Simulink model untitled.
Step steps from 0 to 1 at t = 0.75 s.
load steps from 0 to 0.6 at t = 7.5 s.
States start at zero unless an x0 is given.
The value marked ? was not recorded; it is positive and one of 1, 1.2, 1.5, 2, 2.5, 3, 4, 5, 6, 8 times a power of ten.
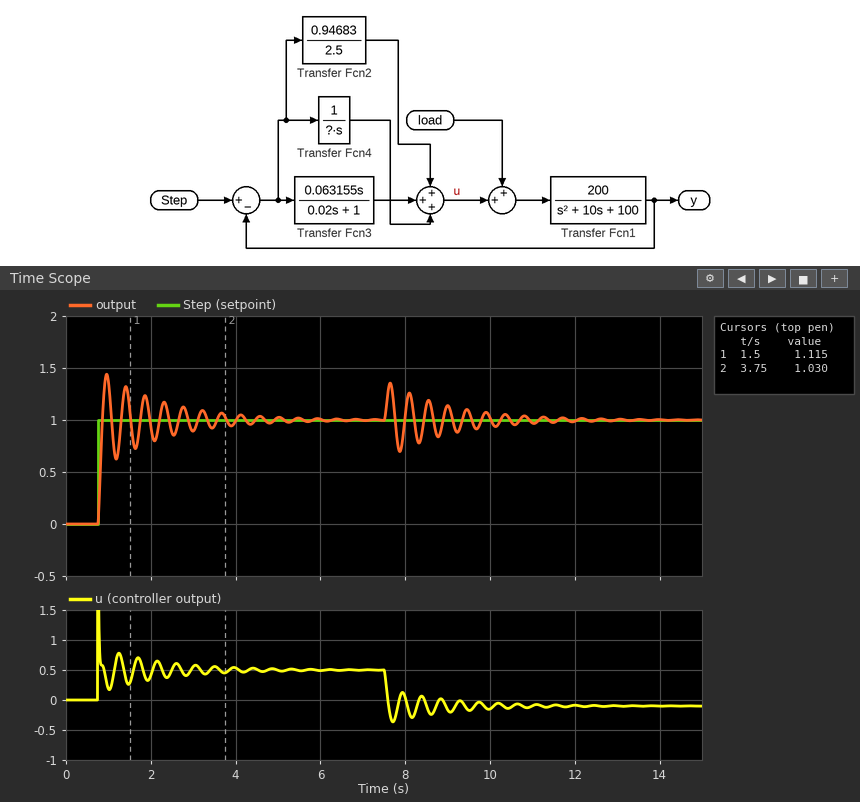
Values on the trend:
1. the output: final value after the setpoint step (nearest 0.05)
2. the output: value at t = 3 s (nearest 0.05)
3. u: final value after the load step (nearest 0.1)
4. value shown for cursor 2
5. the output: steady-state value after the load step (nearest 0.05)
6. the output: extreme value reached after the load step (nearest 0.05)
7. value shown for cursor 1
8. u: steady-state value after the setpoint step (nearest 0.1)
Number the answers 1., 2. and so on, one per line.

1. 1.00
2. 0.90
3. -0.1
4. 1.030
5. 1.00
6. 1.35
7. 1.115
8. 0.5
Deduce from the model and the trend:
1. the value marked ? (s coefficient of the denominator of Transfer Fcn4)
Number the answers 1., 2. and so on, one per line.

1. 0.05
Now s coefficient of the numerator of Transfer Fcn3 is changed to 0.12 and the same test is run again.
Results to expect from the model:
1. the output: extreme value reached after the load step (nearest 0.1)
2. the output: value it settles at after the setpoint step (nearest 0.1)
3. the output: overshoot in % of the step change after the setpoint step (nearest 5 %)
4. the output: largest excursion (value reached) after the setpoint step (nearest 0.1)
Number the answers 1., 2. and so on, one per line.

1. 1.3
2. 1.0
3. 15 %
4. 1.2
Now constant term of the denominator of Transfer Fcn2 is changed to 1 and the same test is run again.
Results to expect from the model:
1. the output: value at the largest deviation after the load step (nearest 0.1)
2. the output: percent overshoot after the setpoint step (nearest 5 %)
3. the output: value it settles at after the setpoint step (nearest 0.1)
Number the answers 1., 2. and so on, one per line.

1. 1.3
2. 35 %
3. 1.0
